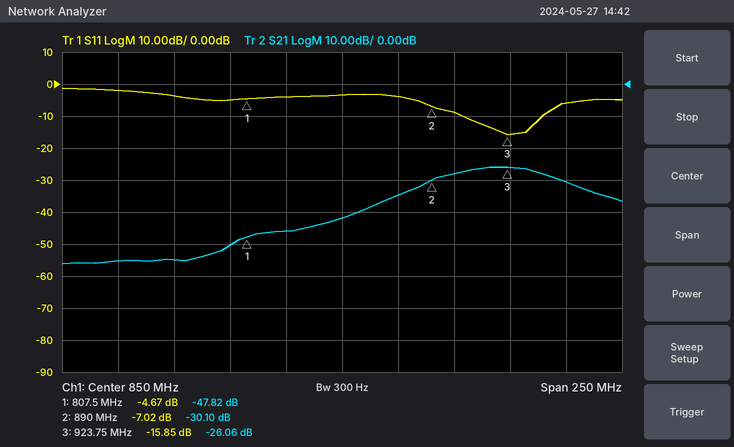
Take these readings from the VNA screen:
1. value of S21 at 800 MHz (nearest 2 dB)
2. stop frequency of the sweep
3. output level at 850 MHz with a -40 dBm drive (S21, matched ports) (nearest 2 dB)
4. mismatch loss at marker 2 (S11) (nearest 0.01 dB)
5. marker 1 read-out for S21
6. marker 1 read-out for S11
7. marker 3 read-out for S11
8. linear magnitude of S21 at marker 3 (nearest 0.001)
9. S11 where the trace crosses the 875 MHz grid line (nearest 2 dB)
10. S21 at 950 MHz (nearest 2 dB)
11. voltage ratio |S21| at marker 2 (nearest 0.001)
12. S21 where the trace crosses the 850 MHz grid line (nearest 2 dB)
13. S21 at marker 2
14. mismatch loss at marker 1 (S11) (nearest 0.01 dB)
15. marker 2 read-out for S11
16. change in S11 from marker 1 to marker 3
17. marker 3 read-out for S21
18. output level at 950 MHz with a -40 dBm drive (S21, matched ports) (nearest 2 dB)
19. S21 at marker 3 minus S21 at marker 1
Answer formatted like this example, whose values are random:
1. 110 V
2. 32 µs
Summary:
1. -50 dB
2. 975 MHz
3. -82 dBm
4. 0.96 dB
5. -47.82 dB
6. -4.67 dB
7. -15.85 dB
8. 0.050
9. -4 dB
10. -30 dB
11. 0.031
12. -42 dB
13. -30.10 dB
14. 1.81 dB
15. -7.02 dB
16. -11.18 dB
17. -26.06 dB
18. -70 dBm
19. 21.76 dB
